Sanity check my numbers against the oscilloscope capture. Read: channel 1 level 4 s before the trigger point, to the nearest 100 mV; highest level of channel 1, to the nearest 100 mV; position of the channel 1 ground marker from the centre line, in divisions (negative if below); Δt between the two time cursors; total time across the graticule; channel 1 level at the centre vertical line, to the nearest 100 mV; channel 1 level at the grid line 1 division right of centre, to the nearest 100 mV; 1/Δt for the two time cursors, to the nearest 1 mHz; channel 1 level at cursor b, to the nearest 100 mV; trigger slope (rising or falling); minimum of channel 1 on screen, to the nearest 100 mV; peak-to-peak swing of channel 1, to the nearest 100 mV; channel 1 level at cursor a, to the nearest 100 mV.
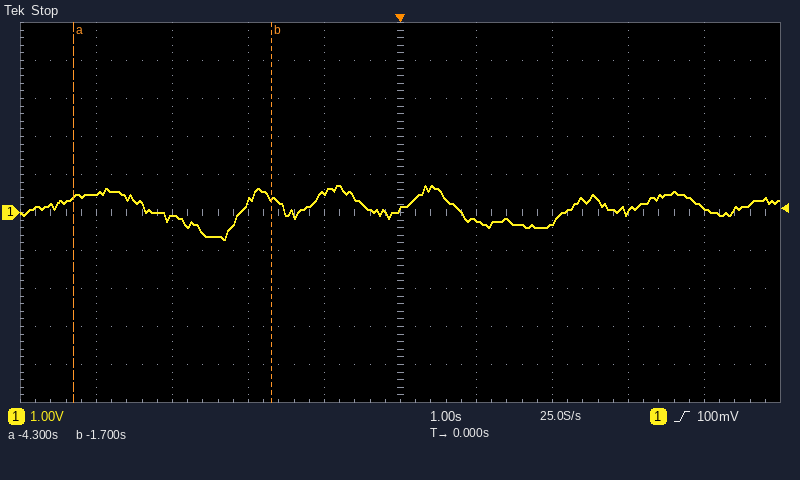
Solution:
500 mV
700 mV
0.0 div
2.6 s
10 s
100 mV
-200 mV
385 mHz
400 mV
rising
-700 mV
1.4 V
400 mV
